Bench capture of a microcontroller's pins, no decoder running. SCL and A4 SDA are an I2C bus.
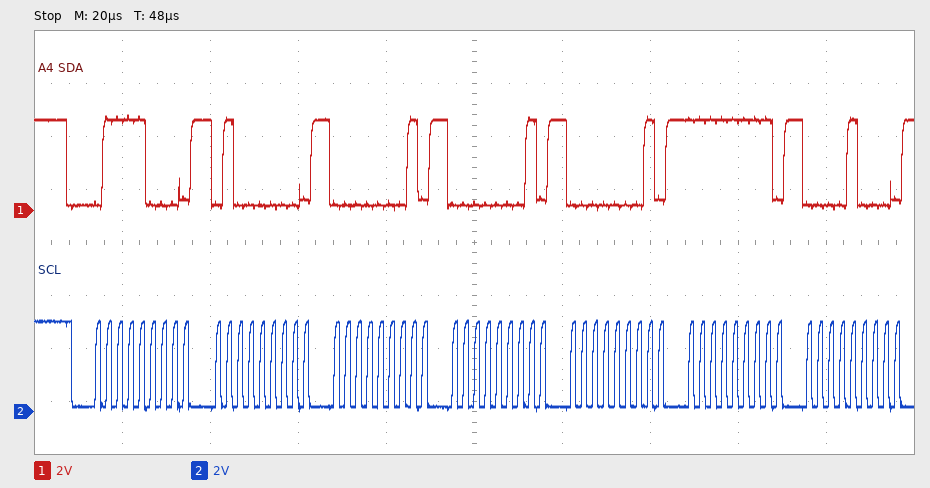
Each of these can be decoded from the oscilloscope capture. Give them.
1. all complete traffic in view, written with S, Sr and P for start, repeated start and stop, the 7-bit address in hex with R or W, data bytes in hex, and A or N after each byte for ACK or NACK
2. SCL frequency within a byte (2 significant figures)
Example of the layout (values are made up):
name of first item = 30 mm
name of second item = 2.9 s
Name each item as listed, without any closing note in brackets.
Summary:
all complete traffic in view, written with S, Sr and P for start, repeated start and stop, the 7-bit address in hex with R or W, data bytes in hex, and A or N after each byte for ACK or NACK = S 3CW A 40 A 01 A 01 A 01 A FF A 08 A
SCL frequency within a byte = 400 kHz
